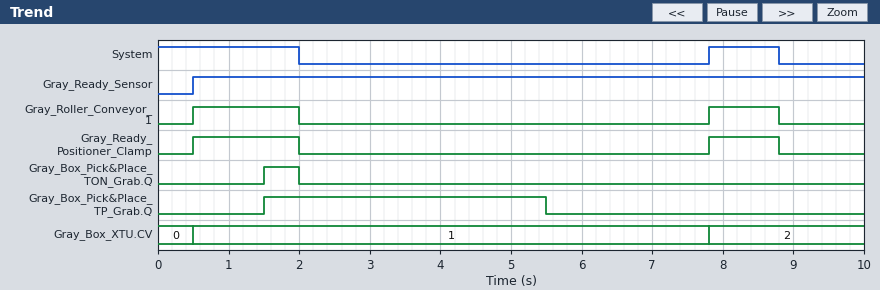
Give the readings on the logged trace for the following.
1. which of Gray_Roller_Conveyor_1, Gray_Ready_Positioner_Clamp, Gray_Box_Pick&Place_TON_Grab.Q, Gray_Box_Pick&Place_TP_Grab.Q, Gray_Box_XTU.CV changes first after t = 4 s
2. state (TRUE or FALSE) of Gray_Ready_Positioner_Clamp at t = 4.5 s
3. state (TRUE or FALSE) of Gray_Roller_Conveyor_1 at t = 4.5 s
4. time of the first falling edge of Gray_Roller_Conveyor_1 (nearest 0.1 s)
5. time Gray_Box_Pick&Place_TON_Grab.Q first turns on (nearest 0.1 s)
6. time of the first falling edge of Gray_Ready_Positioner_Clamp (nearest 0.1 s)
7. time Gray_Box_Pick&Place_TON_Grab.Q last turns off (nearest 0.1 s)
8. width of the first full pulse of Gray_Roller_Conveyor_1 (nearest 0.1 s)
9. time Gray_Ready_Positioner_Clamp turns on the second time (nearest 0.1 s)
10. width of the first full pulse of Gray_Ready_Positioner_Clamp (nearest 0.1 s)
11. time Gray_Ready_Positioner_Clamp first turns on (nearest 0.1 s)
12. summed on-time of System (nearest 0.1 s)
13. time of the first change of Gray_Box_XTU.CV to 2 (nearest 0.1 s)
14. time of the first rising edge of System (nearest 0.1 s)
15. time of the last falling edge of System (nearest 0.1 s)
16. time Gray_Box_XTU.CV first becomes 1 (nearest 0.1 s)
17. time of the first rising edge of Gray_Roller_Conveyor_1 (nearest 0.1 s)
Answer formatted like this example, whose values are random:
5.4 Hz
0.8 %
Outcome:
Gray_Box_Pick&Place_TP_Grab.Q
FALSE
FALSE
2.0 s
1.5 s
2.0 s
2.0 s
1.5 s
7.8 s
1.5 s
0.5 s
3.0 s
7.8 s
7.8 s
8.8 s
0.5 s
0.5 s
